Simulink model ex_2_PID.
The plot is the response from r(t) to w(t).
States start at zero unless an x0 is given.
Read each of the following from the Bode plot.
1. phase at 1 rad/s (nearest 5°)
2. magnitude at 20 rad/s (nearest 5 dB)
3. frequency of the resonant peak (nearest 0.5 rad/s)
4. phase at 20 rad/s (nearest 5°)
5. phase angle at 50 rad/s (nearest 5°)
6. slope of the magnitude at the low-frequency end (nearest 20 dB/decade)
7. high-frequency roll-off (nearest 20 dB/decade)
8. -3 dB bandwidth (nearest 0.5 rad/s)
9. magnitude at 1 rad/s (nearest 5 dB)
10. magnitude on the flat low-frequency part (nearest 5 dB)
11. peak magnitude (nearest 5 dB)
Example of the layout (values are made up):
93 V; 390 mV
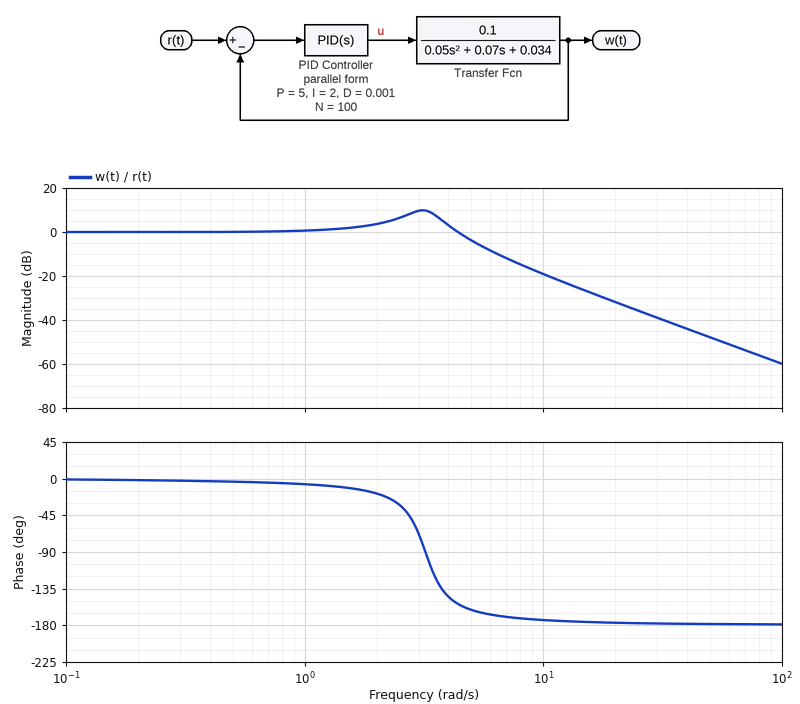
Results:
-5°; -30 dB; 3.0 rad/s; -175°; -180°; 0 dB/decade; -40 dB/decade; 5.0 rad/s; 0 dB; 0 dB; 10 dB
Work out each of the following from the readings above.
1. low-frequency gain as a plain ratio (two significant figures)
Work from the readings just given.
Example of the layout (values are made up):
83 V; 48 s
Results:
1.0
